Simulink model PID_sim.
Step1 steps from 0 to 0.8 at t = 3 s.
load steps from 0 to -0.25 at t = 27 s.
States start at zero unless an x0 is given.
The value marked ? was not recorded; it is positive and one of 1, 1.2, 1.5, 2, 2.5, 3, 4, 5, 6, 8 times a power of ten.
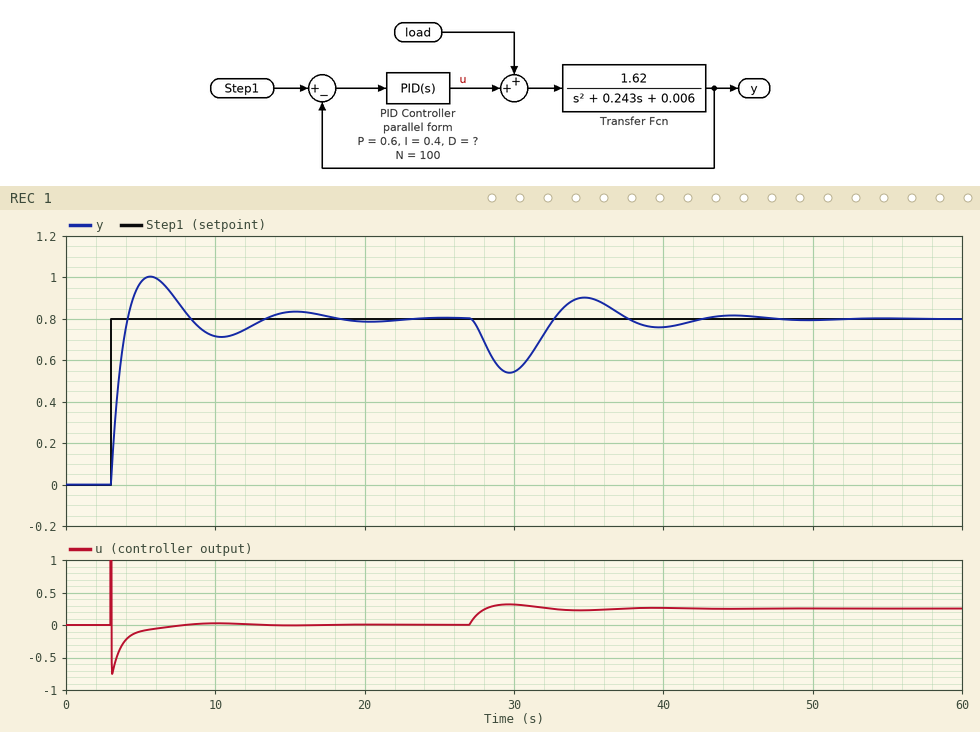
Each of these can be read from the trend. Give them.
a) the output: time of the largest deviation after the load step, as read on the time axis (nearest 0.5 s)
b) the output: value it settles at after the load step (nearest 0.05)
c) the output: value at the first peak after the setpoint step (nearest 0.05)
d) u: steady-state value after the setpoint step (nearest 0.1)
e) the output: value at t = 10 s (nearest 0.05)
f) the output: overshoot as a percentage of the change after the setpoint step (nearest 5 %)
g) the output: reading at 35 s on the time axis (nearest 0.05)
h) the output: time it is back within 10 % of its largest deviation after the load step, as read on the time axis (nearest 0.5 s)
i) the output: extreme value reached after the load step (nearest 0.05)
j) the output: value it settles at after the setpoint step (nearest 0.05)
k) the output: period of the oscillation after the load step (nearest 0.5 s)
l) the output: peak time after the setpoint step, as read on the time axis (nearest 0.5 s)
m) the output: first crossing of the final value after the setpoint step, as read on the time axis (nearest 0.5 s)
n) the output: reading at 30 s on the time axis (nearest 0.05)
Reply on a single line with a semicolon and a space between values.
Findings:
29.5 s; 0.80; 1.00; 0.0; 0.70; 25 %; 0.90; 41.0 s; 0.55; 0.80; 10.0 s; 5.5 s; 4.0 s; 0.55
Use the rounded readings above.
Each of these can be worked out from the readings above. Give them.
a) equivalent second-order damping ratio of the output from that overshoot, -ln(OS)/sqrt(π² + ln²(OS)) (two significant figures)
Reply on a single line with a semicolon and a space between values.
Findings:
0.40
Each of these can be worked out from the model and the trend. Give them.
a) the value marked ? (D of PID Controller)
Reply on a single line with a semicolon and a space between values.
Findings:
1
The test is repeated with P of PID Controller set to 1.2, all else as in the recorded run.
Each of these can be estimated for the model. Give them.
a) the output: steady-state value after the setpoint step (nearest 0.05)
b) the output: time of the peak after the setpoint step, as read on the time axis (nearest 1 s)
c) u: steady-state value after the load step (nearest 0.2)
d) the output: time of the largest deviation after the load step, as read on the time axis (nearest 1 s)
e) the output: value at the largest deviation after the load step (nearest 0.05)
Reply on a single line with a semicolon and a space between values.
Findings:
0.80; 5 s; 0.2; 29 s; 0.60
